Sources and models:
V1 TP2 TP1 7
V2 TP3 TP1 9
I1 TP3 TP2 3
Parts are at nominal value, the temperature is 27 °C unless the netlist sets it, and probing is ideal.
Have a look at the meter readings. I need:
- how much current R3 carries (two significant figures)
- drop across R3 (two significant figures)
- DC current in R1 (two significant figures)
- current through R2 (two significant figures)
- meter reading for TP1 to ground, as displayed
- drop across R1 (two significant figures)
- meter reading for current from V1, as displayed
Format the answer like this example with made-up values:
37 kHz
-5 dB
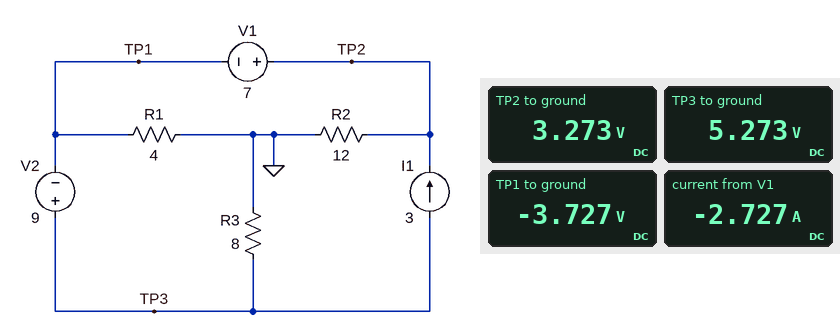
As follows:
660 mA
5.3 V
930 mA
270 mA
-3.727 V
3.7 V
-2.727 A
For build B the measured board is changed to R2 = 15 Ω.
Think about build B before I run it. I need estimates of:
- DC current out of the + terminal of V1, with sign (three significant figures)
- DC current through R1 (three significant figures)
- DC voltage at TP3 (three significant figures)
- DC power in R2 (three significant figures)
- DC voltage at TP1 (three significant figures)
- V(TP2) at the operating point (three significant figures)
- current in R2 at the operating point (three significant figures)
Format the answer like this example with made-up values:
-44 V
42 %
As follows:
-2.77 A
901 mA
5.40 V
769 mW
-3.60 V
3.40 V
226 mA
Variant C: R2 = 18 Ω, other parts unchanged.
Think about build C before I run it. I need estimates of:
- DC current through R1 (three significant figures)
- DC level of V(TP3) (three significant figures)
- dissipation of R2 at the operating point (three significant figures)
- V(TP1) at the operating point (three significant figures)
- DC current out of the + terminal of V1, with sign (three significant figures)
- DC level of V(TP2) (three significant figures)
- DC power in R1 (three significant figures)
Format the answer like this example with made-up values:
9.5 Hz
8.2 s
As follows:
879 mA
5.48 V
674 mW
-3.52 V
-2.81 A
3.48 V
3.09 W
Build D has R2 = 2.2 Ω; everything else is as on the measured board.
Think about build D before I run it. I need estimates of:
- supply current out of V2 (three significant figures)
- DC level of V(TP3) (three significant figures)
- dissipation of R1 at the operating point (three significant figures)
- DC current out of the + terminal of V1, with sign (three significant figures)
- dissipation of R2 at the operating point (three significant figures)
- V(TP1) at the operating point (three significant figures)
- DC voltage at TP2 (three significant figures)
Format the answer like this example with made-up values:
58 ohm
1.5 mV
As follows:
3.48 A
3.81 V
6.74 W
-2.18 A
1.49 W
-5.19 V
1.81 V
